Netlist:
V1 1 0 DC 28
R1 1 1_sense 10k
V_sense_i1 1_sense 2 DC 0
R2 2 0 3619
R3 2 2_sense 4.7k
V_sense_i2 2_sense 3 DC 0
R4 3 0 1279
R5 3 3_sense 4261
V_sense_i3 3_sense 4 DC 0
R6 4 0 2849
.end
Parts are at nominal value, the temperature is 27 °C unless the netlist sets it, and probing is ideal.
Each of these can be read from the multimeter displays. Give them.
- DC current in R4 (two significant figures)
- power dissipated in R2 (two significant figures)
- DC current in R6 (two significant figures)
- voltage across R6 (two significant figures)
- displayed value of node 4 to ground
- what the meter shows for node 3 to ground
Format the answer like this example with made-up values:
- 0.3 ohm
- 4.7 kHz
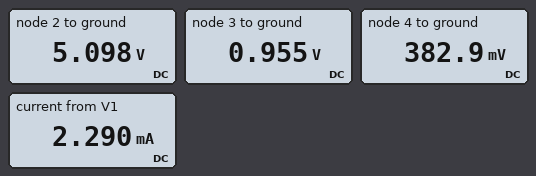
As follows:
- 750 µA
- 7.2 mW
- 130 µA
- 380 mV
- 382.9 mV
- 0.955 V
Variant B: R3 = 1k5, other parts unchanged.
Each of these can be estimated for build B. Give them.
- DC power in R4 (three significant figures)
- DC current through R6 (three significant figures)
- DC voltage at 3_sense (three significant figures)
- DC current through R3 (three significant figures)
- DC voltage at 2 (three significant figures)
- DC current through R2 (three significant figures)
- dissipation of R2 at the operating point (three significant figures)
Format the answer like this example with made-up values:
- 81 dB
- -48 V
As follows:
- 1.85 mW
- 216 µA
- 617 mV
- 1.42 mA
- 3.67 V
- 1.01 mA
- 3.72 mW
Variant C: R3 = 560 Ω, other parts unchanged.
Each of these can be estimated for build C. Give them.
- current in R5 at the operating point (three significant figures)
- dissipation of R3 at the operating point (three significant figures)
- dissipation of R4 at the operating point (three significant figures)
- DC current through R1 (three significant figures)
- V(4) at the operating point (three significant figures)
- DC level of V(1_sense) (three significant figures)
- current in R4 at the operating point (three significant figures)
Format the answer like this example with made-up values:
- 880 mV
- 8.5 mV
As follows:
- 264 µA
- 1.68 mW
- 2.75 mW
- 2.52 mA
- 751 mV
- 2.84 V
- 1.47 mA
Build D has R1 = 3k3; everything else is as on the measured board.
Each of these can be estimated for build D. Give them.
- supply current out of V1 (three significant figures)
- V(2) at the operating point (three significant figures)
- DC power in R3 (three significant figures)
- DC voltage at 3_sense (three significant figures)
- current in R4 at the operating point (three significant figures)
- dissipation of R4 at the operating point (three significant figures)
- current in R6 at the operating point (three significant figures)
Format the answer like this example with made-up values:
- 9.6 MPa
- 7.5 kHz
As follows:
- 5.07 mA
- 11.3 V
- 17.9 mW
- 847 mV
- 1.65 mA
- 3.49 mW
- 297 µA
